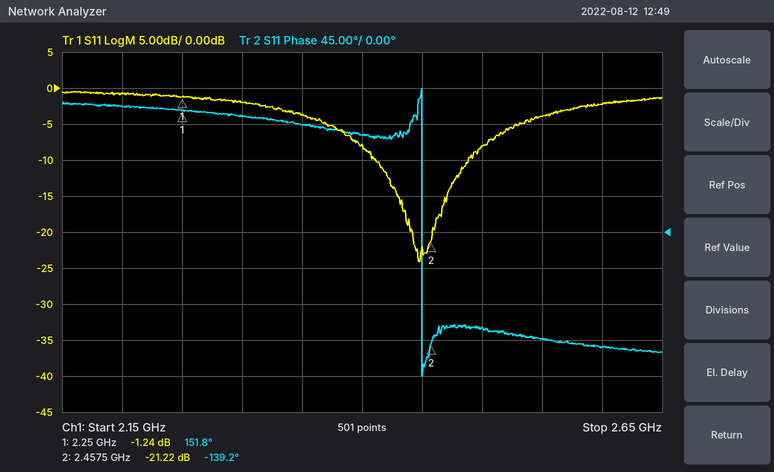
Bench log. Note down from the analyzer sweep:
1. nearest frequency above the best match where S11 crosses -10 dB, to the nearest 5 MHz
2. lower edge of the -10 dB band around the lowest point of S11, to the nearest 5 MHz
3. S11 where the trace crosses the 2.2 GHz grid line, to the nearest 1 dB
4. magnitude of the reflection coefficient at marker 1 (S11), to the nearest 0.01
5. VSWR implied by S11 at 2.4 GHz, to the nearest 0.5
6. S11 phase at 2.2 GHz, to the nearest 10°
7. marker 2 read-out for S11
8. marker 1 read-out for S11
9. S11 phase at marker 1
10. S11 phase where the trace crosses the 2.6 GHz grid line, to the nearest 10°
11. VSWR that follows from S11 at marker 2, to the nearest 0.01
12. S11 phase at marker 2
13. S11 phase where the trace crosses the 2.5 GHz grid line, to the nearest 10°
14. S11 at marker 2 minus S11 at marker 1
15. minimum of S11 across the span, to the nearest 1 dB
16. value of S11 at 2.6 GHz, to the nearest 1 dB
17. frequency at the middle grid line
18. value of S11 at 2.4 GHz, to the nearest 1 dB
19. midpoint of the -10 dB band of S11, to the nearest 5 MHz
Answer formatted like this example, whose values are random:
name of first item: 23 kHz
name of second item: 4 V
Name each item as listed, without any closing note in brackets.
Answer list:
nearest frequency above the best match where S11 crosses -10 dB, to the nearest 5 MHz: 2.490 GHz
lower edge of the -10 dB band around the lowest point of S11, to the nearest 5 MHz: 2.410 GHz
S11 where the trace crosses the 2.2 GHz grid line, to the nearest 1 dB: -1 dB
magnitude of the reflection coefficient at marker 1 (S11), to the nearest 0.01: 0.87
VSWR implied by S11 at 2.4 GHz, to the nearest 0.5: 2.5
S11 phase at 2.2 GHz, to the nearest 10°: 160°
marker 2 read-out for S11: -21.22 dB
marker 1 read-out for S11: -1.24 dB
S11 phase at marker 1: 151.8°
S11 phase where the trace crosses the 2.6 GHz grid line, to the nearest 10°: -140°
VSWR that follows from S11 at marker 2, to the nearest 0.01: 1.19
S11 phase at marker 2: -139.2°
S11 phase where the trace crosses the 2.5 GHz grid line, to the nearest 10°: -120°
S11 at marker 2 minus S11 at marker 1: -19.98 dB
minimum of S11 across the span, to the nearest 1 dB: -24 dB
value of S11 at 2.6 GHz, to the nearest 1 dB: -2 dB
frequency at the middle grid line: 2.4 GHz
value of S11 at 2.4 GHz, to the nearest 1 dB: -8 dB
midpoint of the -10 dB band of S11, to the nearest 5 MHz: 2.450 GHz
